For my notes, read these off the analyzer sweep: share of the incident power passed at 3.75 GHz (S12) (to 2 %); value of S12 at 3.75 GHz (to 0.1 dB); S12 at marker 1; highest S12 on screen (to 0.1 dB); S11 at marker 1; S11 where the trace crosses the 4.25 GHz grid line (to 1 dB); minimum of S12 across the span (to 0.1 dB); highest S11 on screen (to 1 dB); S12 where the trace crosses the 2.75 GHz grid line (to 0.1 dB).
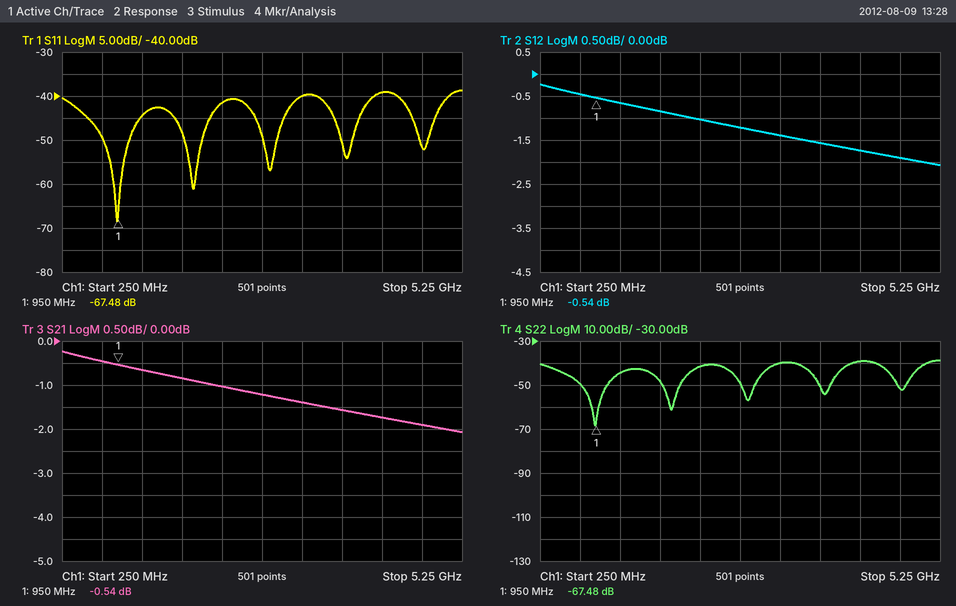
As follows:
70 %
-1.6 dB
-0.54 dB
-0.2 dB
-67.48 dB
-39 dB
-2.1 dB
-39 dB
-1.2 dB
